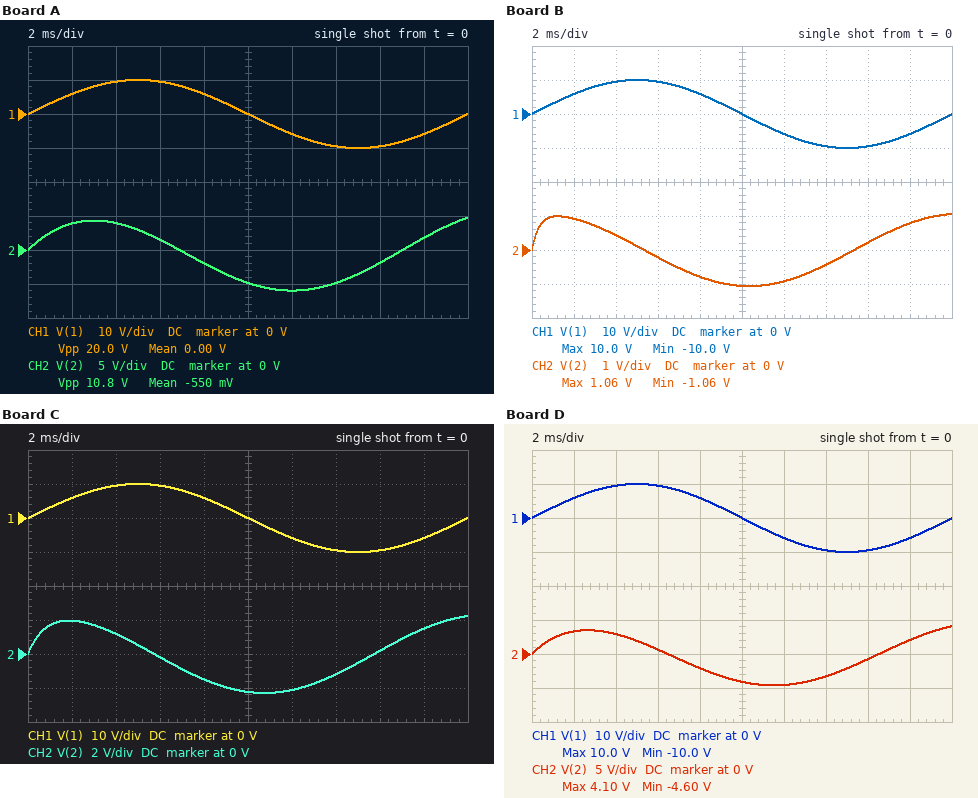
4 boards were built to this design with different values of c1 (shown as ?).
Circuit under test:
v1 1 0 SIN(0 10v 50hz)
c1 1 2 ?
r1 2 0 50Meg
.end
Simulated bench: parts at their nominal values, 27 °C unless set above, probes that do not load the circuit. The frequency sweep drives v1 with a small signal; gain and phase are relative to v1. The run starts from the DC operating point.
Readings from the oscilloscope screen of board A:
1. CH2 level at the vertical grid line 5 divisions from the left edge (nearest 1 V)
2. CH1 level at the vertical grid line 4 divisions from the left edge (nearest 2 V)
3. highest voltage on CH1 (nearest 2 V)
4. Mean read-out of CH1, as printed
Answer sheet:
-5 V
6 V
10 V
0.00 V
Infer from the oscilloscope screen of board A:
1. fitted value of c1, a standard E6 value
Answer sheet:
47 pF
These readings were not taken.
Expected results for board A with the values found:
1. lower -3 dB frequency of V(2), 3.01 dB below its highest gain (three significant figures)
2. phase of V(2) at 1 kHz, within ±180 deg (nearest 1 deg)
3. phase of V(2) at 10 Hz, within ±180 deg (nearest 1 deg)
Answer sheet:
67.7 Hz
4 deg
82 deg
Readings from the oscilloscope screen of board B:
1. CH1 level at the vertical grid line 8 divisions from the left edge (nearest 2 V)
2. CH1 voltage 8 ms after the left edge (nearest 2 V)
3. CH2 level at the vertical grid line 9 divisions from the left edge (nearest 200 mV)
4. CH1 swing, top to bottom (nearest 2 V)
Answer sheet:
-10 V
6 V
800 mV
20 V
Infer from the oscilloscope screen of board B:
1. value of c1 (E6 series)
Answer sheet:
6.8 pF
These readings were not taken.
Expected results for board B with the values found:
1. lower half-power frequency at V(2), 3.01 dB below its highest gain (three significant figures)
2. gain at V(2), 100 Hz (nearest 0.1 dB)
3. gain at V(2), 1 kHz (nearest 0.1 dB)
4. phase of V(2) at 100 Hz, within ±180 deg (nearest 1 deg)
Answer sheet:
468 Hz
-13.6 dB
-0.9 dB
78 deg
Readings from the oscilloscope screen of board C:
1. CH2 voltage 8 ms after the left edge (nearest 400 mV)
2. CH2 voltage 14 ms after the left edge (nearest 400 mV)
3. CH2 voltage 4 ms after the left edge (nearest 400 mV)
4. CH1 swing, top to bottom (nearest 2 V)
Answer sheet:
-1.6 V
-1.2 V
1.2 V
20 V
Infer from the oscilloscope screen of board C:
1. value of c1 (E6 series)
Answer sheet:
15 pF
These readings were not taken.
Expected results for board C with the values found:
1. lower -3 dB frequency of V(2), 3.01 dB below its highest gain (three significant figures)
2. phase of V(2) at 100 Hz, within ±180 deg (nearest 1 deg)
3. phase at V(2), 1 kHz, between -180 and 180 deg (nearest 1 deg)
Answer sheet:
212 Hz
65 deg
12 deg
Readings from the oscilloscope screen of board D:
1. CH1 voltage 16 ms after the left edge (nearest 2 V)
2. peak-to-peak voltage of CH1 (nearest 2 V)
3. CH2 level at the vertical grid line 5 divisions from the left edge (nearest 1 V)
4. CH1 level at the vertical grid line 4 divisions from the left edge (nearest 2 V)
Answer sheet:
-10 V
20 V
-4 V
6 V
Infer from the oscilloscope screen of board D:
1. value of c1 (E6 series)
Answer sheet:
33 pF
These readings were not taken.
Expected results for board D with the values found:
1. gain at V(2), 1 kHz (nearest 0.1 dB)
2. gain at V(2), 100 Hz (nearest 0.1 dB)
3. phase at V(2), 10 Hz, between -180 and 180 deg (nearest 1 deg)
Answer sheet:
0 dB
-2.9 dB
84 deg
